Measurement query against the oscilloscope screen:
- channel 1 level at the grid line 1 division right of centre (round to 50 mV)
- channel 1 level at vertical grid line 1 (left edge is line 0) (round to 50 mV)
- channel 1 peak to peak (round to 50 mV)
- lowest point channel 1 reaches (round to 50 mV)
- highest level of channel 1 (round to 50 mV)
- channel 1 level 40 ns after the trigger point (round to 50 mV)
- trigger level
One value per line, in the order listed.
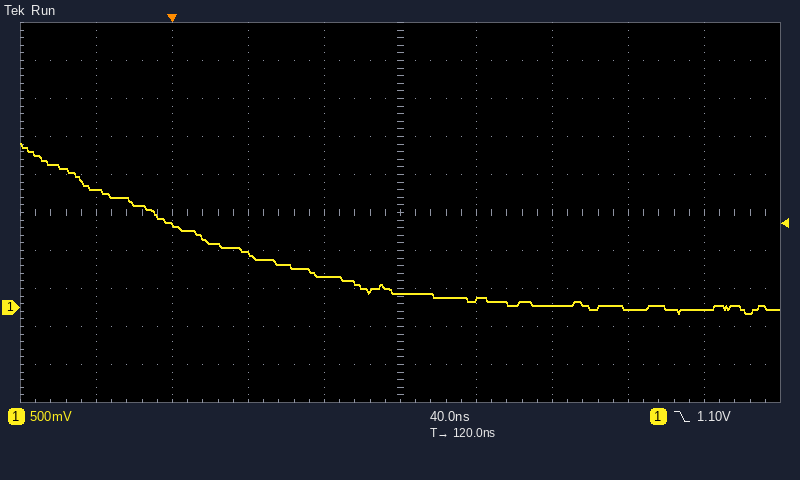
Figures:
100 mV
1.55 V
2.25 V
-100 mV
2.15 V
700 mV
1.10 V
